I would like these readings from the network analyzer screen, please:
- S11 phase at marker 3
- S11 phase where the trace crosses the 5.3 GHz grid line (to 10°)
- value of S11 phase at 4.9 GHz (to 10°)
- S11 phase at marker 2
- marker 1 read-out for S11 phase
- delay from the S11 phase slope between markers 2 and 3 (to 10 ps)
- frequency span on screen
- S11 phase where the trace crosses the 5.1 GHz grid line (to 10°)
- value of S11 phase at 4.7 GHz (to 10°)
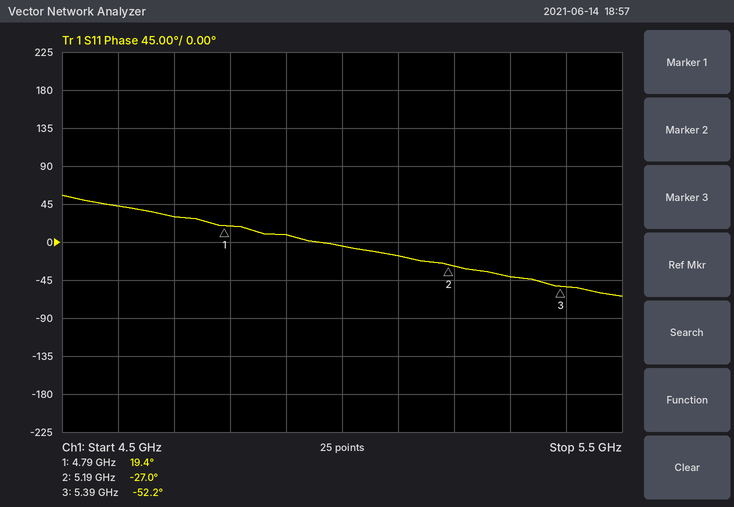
-52.2°
-40°
10°
-27.0°
19.4°
350 ps
1 GHz
-20°
30°
